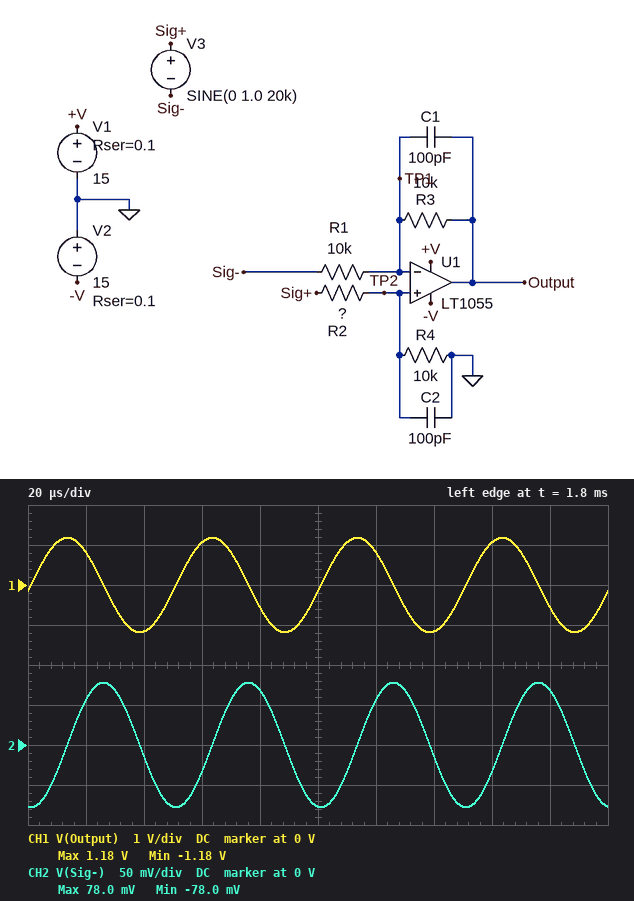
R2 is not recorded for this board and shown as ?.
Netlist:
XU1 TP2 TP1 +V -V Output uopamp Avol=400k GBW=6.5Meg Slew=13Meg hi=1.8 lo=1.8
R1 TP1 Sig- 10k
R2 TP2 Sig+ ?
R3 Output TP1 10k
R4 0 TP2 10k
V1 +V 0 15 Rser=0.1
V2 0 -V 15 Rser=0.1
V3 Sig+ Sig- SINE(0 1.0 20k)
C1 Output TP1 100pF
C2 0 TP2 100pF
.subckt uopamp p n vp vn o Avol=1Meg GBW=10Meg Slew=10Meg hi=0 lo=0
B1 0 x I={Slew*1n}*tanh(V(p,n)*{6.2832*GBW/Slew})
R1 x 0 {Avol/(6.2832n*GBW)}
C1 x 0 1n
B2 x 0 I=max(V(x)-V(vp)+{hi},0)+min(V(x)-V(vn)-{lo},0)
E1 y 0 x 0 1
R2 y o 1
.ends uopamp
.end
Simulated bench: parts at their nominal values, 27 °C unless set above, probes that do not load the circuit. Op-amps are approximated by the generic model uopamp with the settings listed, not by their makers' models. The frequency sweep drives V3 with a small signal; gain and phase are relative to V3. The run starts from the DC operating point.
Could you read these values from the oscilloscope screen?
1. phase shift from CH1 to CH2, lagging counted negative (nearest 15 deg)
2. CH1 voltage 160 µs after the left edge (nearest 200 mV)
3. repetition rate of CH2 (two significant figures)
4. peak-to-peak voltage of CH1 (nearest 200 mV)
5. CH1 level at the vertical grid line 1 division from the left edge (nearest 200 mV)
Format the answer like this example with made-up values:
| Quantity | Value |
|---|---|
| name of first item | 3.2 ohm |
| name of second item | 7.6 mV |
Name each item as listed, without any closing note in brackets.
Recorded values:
| Quantity | Value |
|---|---|
| phase shift from CH1 to CH2, lagging counted negative | -90 deg |
| CH1 voltage 160 µs after the left edge | 1.0 V |
| repetition rate of CH2 | 20 kHz |
| peak-to-peak voltage of CH1 | 2.4 V |
| CH1 level at the vertical grid line 1 division from the left edge | 800 mV |
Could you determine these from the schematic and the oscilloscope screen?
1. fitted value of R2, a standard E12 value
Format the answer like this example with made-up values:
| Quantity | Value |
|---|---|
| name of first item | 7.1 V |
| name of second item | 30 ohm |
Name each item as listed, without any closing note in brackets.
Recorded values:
| Quantity | Value |
|---|---|
| fitted value of R2, a standard E12 value | 6.8 kΩ |
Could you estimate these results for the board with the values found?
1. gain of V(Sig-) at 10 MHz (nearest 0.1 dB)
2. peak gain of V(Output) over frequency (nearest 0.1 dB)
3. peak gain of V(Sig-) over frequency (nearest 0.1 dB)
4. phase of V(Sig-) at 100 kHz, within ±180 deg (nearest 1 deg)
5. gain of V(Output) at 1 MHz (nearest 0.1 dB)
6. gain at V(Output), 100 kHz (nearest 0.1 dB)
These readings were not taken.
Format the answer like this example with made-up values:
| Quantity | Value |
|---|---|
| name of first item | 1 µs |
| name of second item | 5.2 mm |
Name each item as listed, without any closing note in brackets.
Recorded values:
| Quantity | Value |
|---|---|
| gain of V(Sig-) at 10 MHz | -4.5 dB |
| peak gain of V(Output) over frequency | 1.5 dB |
| peak gain of V(Sig-) over frequency | -4.4 dB |
| phase of V(Sig-) at 100 kHz, within ±180 deg | -123 deg |
| gain of V(Output) at 1 MHz | -14.9 dB |
| gain at V(Output), 100 kHz | 0 dB |
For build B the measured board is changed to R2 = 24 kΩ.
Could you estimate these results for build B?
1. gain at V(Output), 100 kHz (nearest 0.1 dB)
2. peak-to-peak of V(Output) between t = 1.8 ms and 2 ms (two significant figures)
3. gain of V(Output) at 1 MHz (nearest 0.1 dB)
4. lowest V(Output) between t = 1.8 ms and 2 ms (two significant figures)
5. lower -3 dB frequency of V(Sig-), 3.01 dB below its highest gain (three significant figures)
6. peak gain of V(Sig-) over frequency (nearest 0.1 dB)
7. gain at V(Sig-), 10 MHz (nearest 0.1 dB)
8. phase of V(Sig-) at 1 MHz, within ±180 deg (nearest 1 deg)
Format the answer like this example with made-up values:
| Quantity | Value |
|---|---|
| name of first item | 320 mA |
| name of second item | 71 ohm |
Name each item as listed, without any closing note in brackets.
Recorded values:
| Quantity | Value |
|---|---|
| gain at V(Output), 100 kHz | -6.1 dB |
| peak-to-peak of V(Output) between t = 1.8 ms and 2 ms | 1.2 V |
| gain of V(Output) at 1 MHz | -20.9 dB |
| lowest V(Output) between t = 1.8 ms and 2 ms | -580 mV |
| lower -3 dB frequency of V(Sig-), 3.01 dB below its highest gain | 155 kHz |
| peak gain of V(Sig-) over frequency | -10.4 dB |
| gain at V(Sig-), 10 MHz | -10.5 dB |
| phase of V(Sig-) at 1 MHz, within ±180 deg | -171 deg |
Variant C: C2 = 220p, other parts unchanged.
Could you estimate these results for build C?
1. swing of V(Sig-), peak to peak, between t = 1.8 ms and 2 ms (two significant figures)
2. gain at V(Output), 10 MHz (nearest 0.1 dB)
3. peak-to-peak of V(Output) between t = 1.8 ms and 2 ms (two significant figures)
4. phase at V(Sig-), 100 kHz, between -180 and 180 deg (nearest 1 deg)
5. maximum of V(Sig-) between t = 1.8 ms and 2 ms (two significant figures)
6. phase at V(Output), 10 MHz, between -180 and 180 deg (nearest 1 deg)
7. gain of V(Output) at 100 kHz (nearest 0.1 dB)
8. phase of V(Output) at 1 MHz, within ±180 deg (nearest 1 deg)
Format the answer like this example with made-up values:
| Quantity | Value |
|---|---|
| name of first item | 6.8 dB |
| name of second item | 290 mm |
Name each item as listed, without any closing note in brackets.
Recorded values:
| Quantity | Value |
|---|---|
| swing of V(Sig-), peak to peak, between t = 1.8 ms and 2 ms | 320 mV |
| gain at V(Output), 10 MHz | -42.5 dB |
| peak-to-peak of V(Output) between t = 1.8 ms and 2 ms | 2.3 V |
| phase at V(Sig-), 100 kHz, between -180 and 180 deg | -144 deg |
| maximum of V(Sig-) between t = 1.8 ms and 2 ms | 160 mV |
| phase at V(Output), 10 MHz, between -180 and 180 deg | -146 deg |
| gain of V(Output) at 100 kHz | -1.6 dB |
| phase of V(Output) at 1 MHz, within ±180 deg | -91 deg |
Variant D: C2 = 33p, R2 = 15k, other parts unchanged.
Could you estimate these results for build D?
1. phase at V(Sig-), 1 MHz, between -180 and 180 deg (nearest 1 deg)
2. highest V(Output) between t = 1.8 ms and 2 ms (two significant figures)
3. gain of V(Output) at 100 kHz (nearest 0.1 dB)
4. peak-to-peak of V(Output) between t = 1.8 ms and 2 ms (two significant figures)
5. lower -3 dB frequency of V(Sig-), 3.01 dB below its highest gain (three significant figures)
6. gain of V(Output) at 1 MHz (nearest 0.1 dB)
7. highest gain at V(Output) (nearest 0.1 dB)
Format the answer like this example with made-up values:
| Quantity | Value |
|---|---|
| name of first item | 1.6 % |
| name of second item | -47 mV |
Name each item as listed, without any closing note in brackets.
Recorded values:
| Quantity | Value |
|---|---|
| phase at V(Sig-), 1 MHz, between -180 and 180 deg | -156 deg |
| highest V(Output) between t = 1.8 ms and 2 ms | 800 mV |
| gain of V(Output) at 100 kHz | -2.9 dB |
| peak-to-peak of V(Output) between t = 1.8 ms and 2 ms | 1.6 V |
| lower -3 dB frequency of V(Sig-), 3.01 dB below its highest gain | 445 kHz |
| gain of V(Output) at 1 MHz | -13.0 dB |
| highest gain at V(Output) | -1.9 dB |
